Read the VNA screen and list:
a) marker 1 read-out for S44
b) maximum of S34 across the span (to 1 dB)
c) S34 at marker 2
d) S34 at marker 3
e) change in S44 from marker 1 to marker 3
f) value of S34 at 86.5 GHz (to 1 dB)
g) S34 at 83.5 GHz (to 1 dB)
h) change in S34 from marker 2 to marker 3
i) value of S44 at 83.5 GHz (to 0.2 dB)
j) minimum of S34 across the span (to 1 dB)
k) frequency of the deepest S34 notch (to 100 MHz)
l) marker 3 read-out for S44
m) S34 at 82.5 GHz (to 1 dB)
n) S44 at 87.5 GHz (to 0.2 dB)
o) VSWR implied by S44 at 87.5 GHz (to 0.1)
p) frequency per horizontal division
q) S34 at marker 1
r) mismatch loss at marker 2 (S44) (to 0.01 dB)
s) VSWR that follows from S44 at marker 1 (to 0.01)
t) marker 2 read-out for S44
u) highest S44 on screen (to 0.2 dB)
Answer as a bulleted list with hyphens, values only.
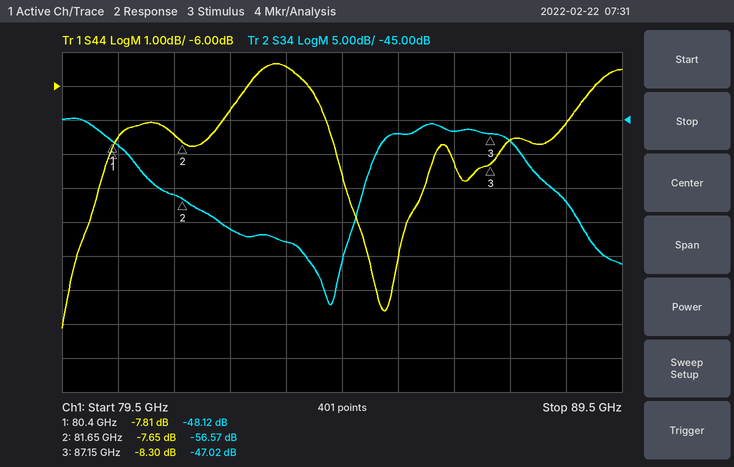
- -7.81 dB
- -45 dB
- -56.57 dB
- -47.02 dB
- -0.49 dB
- -47 dB
- -63 dB
- 9.55 dB
- -5.4 dB
- -72 dB
- 84.3 GHz
- -8.30 dB
- -61 dB
- -7.6 dB
- 2.4
- 1 GHz
- -48.12 dB
- 0.82 dB
- 2.37
- -7.65 dB
- -5.4 dB
